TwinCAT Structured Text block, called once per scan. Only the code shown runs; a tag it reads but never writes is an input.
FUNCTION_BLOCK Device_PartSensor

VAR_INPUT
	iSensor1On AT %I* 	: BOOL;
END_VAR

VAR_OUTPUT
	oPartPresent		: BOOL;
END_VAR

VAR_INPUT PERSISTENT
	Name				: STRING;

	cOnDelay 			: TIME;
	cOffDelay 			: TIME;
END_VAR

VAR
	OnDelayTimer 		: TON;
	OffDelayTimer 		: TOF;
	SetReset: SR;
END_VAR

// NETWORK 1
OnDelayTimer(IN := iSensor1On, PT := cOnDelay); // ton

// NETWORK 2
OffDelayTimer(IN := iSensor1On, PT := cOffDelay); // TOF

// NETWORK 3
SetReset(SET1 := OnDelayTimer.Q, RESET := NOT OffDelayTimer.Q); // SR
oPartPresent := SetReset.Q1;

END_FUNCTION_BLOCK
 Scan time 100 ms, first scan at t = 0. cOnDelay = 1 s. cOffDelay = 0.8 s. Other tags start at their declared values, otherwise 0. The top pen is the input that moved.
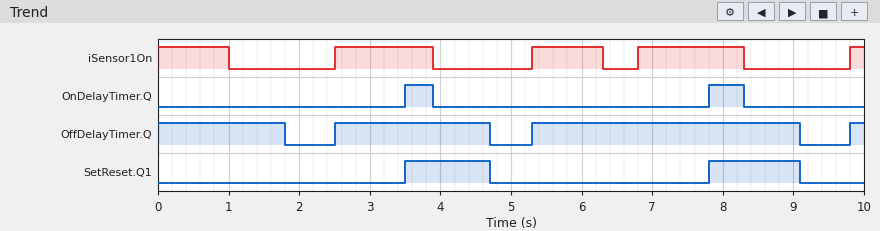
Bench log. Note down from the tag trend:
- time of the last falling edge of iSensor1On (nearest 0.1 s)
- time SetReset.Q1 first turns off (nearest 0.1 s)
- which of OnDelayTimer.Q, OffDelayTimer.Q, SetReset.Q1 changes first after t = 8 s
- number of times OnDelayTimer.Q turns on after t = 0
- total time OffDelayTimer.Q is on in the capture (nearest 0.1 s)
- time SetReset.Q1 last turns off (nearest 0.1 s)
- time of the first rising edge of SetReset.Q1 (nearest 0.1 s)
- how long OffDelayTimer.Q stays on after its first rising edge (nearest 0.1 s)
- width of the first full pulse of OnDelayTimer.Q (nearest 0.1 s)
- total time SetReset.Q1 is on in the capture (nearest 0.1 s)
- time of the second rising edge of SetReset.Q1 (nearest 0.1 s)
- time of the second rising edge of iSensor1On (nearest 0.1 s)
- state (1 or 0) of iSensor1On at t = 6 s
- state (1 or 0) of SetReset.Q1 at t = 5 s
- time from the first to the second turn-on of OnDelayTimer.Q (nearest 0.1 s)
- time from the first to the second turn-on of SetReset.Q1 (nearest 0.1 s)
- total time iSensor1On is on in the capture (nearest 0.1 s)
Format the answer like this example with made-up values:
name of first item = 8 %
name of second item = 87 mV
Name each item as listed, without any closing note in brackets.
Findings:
time of the last falling edge of iSensor1On = 8.3 s
time SetReset.Q1 first turns off = 4.7 s
which of OnDelayTimer.Q, OffDelayTimer.Q, SetReset.Q1 changes first after t = 8 s = OnDelayTimer.Q
number of times OnDelayTimer.Q turns on after t = 0 = 2
total time OffDelayTimer.Q is on in the capture = 8.0 s
time SetReset.Q1 last turns off = 9.1 s
time of the first rising edge of SetReset.Q1 = 3.5 s
how long OffDelayTimer.Q stays on after its first rising edge = 2.2 s
width of the first full pulse of OnDelayTimer.Q = 0.4 s
total time SetReset.Q1 is on in the capture = 2.5 s
time of the second rising edge of SetReset.Q1 = 7.8 s
time of the second rising edge of iSensor1On = 5.3 s
state (1 or 0) of iSensor1On at t = 6 s = 1
state (1 or 0) of SetReset.Q1 at t = 5 s = 0
time from the first to the second turn-on of OnDelayTimer.Q = 4.3 s
time from the first to the second turn-on of SetReset.Q1 = 4.3 s
total time iSensor1On is on in the capture = 5.1 s
